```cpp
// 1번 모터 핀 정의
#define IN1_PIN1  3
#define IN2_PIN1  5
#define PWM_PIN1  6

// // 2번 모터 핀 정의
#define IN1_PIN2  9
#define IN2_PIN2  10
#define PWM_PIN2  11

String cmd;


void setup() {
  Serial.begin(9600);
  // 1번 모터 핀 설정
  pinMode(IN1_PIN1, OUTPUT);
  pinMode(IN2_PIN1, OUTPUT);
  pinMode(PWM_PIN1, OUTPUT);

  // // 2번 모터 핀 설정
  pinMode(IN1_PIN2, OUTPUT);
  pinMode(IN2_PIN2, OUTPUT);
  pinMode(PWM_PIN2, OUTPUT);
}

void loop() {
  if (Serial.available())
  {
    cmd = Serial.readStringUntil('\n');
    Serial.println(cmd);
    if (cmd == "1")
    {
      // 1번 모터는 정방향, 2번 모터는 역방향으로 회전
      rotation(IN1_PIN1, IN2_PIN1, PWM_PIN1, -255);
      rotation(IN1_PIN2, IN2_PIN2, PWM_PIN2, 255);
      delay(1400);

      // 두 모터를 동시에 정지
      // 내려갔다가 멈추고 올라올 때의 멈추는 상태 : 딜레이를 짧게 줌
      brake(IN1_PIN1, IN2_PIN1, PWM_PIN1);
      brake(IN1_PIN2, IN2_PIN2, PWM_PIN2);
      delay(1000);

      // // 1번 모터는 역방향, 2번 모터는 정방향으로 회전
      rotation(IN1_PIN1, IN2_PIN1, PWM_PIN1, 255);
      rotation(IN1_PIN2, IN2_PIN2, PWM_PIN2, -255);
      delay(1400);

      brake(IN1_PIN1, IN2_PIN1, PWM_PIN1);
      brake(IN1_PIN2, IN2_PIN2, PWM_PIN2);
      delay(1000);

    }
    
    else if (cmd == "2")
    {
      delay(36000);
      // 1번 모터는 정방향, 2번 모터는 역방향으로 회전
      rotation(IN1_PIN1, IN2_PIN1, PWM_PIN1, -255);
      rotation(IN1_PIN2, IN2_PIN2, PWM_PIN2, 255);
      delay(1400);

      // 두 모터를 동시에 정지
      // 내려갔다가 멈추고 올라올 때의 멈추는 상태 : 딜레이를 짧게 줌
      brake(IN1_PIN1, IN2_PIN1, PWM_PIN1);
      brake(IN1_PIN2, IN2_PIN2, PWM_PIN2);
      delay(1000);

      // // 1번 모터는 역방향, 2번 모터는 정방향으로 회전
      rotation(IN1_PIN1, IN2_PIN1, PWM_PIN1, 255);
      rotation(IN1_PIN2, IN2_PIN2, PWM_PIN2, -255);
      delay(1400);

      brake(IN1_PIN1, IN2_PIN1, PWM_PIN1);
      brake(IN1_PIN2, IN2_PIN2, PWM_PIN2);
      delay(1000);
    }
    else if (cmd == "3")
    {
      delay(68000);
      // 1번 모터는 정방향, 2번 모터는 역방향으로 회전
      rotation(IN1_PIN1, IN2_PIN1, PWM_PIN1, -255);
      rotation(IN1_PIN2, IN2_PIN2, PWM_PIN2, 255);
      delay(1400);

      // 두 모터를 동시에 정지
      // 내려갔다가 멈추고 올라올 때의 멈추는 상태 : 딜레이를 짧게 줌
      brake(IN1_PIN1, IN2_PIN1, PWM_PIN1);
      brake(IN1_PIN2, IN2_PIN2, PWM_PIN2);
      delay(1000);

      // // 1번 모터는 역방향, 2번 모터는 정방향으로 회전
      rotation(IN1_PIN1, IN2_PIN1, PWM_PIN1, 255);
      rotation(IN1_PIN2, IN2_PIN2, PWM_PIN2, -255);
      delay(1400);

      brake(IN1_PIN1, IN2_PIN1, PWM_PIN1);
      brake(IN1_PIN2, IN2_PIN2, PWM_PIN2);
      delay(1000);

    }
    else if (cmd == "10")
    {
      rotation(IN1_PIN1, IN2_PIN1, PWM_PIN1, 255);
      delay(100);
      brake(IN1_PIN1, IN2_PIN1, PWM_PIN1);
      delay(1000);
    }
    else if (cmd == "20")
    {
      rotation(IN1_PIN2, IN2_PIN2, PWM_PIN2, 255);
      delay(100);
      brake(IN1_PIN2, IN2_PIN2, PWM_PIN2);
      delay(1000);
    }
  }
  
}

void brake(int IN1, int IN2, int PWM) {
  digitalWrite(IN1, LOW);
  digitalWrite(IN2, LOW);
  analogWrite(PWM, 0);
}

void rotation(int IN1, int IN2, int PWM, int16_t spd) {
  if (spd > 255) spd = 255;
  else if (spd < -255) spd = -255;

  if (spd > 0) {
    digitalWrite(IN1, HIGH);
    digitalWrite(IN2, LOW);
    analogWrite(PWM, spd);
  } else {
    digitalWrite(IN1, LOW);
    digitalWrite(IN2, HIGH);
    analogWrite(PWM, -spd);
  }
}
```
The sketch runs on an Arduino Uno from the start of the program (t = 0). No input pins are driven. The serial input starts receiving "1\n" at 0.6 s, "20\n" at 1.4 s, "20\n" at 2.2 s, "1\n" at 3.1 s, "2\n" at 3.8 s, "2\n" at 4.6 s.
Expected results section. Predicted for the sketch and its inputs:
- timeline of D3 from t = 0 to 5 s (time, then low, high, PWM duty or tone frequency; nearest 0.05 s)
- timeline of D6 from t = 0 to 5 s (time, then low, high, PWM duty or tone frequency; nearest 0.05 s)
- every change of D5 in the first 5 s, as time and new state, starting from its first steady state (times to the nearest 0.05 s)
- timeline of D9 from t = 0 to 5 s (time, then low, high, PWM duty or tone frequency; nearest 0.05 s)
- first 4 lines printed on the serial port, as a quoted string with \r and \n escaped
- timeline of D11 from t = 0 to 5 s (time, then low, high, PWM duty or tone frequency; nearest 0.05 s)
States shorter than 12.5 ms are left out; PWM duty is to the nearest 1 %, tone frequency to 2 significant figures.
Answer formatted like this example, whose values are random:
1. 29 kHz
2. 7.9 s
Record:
1. 0 s low; 3 s high; 4.4 s low
2. 0 s low; 0.6 s high; 2 s low; 3 s high; 4.4 s low
3. 0 s low; 0.6 s high; 2 s low
4. 0 s low; 0.6 s high; 2 s low
5. "1\r\n20\r\n20\r\n1\r\n"
6. 0 s low; 0.6 s high; 2 s low; 3 s high; 4.4 s low
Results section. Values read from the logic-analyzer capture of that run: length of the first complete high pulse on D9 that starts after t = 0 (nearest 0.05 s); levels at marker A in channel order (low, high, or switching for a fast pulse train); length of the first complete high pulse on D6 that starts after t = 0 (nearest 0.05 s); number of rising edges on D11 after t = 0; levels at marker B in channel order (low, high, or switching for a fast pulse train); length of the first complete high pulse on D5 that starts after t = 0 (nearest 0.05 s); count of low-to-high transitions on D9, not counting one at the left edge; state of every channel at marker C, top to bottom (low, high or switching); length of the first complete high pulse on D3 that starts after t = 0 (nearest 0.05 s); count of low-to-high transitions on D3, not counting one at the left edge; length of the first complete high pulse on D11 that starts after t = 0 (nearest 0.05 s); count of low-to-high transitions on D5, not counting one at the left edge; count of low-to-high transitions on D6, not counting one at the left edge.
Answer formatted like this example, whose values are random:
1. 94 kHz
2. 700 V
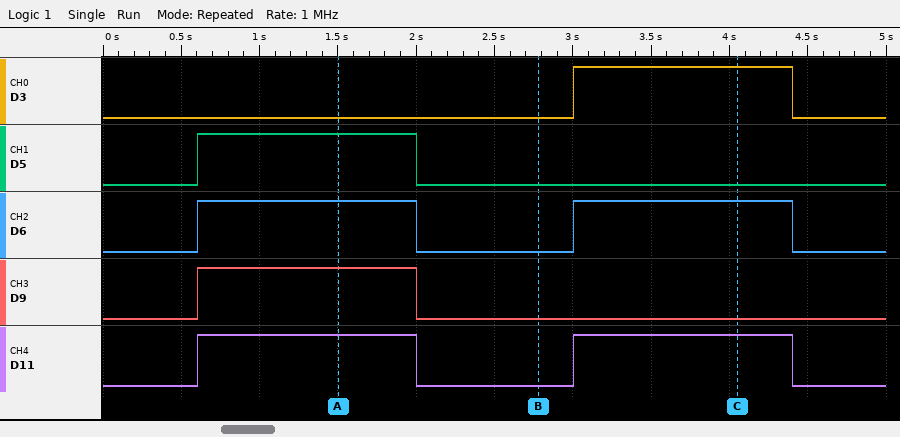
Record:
1. 1.40 s
2. D3 low, D5 high, D6 high, D9 high, D11 high
3. 1.40 s
4. 2
5. D3 low, D5 low, D6 low, D9 low, D11 low
6. 1.40 s
7. 1
8. D3 high, D5 low, D6 high, D9 low, D11 high
9. 1.40 s
10. 1
11. 1.40 s
12. 1
13. 2
